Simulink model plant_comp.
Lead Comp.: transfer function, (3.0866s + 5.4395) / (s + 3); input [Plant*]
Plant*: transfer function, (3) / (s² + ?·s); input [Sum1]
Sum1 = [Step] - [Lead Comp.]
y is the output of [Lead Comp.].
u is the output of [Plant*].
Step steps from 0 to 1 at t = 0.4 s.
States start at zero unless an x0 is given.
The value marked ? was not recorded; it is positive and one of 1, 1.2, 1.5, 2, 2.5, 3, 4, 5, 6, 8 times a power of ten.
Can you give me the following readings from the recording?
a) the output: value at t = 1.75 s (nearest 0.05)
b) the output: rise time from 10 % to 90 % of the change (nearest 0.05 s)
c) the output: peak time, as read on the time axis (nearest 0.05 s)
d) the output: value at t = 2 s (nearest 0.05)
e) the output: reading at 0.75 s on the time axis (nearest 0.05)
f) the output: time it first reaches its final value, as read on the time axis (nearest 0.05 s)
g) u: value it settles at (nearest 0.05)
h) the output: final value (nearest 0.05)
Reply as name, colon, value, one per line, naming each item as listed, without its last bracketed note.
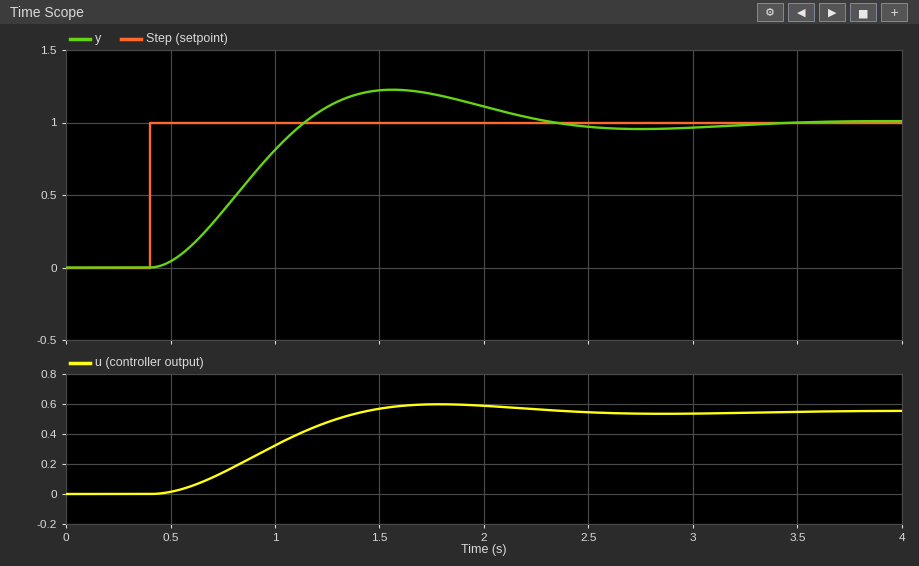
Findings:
the output: value at t = 1.75 s: 1.20
the output: rise time from 10 % to 90 % of the change: 0.50 s
the output: peak time, as read on the time axis: 1.55 s
the output: value at t = 2 s: 1.10
the output: reading at 0.75 s on the time axis: 0.40
the output: time it first reaches its final value, as read on the time axis: 1.15 s
u: value it settles at: 0.55
the output: final value: 1.00
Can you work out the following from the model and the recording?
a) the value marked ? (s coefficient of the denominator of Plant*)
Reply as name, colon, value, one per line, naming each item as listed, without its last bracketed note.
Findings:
the value marked ?: 1.5
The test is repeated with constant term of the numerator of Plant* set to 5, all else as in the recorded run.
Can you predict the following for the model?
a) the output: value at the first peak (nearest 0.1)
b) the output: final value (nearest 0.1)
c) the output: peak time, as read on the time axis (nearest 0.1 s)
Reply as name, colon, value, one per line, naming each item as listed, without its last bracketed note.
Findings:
the output: value at the first peak: 1.3
the output: final value: 1.0
the output: peak time, as read on the time axis: 1.3 s
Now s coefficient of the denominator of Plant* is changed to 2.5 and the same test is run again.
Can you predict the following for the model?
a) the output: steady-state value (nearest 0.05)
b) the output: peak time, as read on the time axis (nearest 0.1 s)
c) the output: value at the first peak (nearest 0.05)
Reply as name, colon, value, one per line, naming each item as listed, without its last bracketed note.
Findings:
the output: steady-state value: 1.00
the output: peak time, as read on the time axis: 1.7 s
the output: value at the first peak: 1.05
